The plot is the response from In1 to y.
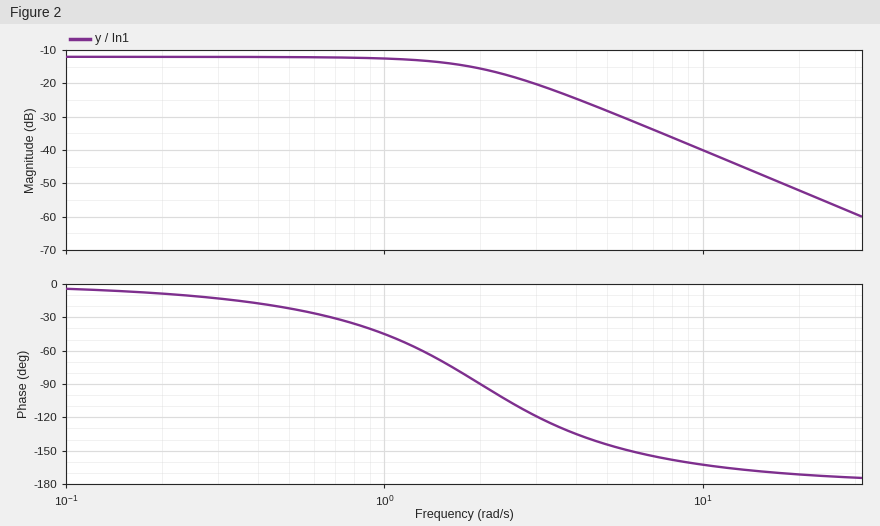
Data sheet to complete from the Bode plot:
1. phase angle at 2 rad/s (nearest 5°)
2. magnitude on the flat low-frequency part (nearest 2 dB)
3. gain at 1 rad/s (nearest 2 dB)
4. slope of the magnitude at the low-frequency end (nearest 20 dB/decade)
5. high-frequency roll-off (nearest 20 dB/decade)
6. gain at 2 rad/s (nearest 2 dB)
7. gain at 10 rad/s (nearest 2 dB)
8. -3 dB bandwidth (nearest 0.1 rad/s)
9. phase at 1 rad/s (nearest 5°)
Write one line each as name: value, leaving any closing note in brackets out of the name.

phase angle at 2 rad/s: -90°
magnitude on the flat low-frequency part: -12 dB
gain at 1 rad/s: -12 dB
slope of the magnitude at the low-frequency end: 0 dB/decade
high-frequency roll-off: -40 dB/decade
gain at 2 rad/s: -16 dB
gain at 10 rad/s: -40 dB
-3 dB bandwidth: 1.9 rad/s
phase at 1 rad/s: -45°
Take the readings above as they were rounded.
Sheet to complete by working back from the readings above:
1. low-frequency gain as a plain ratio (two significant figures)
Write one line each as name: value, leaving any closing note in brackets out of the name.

low-frequency gain as a plain ratio: 0.25
